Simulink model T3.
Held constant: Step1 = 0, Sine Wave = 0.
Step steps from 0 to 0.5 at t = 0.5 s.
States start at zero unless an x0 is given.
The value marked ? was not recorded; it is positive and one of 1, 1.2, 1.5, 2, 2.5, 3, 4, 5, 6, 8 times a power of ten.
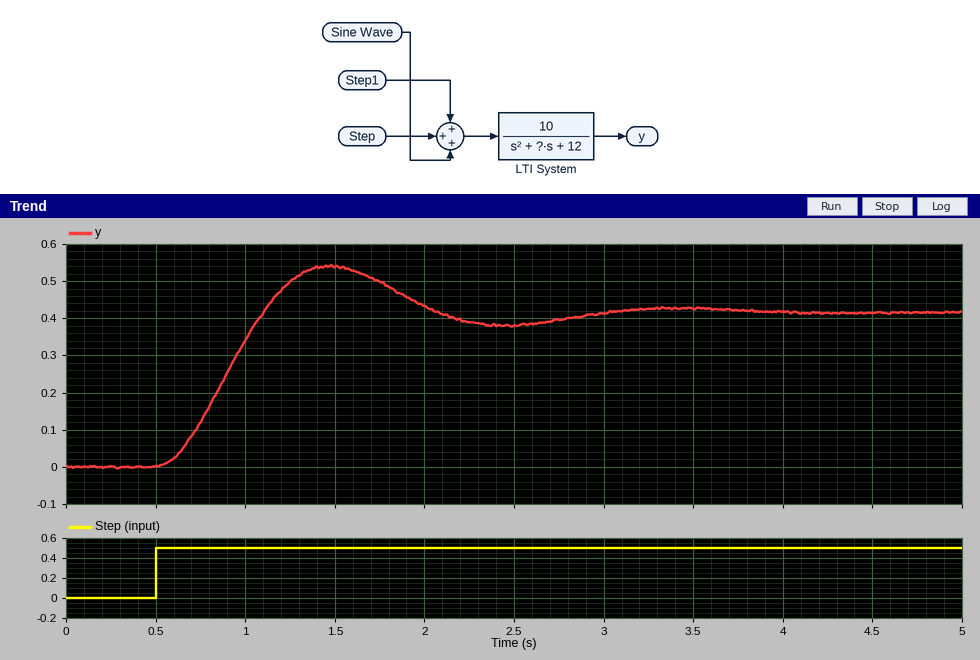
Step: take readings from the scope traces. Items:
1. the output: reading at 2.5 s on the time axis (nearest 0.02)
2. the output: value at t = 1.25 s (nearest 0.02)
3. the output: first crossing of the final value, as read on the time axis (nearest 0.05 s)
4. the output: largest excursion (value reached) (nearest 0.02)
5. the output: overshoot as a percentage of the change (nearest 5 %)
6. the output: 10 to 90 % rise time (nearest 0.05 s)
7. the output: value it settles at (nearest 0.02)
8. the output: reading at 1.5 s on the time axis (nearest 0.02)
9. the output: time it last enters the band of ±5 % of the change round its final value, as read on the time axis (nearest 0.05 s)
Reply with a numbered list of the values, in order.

1. 0.38
2. 0.50
3. 1.10 s
4. 0.54
5. 30 %
6. 0.40 s
7. 0.42
8. 0.54
9. 2.75 s
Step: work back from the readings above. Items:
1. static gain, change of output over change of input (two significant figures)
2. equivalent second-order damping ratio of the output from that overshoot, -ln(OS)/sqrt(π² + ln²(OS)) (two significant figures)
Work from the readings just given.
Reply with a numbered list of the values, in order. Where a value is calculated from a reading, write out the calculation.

1. (0.42 - 0) / (0.5 - 0) = 0.84
2. ln(0.3) = -1.204; 1.204 / sqrt(9.870 + 1.450) = 0.36
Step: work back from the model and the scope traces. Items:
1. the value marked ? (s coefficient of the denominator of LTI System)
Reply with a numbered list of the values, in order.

1. 2.5
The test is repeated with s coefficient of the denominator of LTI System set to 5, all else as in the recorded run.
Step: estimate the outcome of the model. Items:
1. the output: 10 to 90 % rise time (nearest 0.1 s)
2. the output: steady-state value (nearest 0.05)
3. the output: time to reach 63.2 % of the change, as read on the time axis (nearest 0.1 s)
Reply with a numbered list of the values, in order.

1. 0.6 s
2. 0.40
3. 1.0 s
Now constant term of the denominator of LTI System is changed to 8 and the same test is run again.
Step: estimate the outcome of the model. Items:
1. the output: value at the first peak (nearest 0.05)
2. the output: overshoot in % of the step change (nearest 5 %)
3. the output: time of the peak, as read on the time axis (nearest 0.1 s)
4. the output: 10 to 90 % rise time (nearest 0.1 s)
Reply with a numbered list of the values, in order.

1. 0.75
2. 20 %
3. 1.7 s
4. 0.5 s
